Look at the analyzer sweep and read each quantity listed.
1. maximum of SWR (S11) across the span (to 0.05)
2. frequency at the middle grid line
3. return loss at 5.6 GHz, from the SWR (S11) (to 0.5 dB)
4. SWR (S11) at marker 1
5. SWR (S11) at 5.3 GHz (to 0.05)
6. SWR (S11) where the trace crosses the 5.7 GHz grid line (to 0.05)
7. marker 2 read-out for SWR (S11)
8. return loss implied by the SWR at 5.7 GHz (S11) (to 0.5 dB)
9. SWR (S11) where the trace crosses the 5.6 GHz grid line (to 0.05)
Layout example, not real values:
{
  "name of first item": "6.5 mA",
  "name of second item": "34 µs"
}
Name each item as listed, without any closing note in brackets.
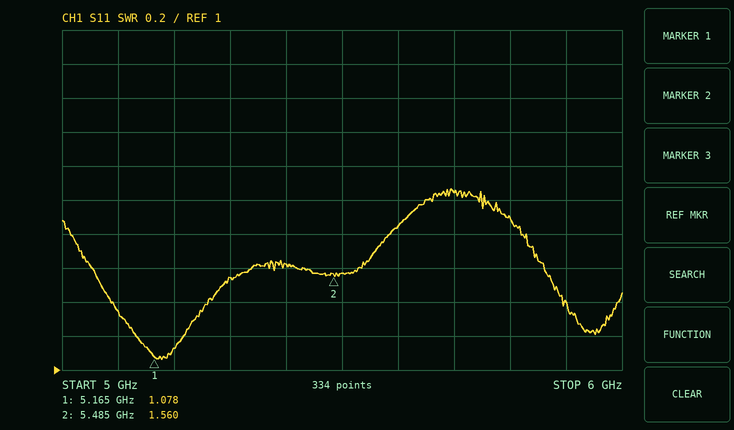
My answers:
{
  "maximum of SWR (S11) across the span": "2.05",
  "frequency at the middle grid line": "5.5 GHz",
  "return loss at 5.6 GHz, from the SWR (S11)": "10.5 dB",
  "SWR (S11) at marker 1": "1.078",
  "SWR (S11) at 5.3 GHz": "1.55",
  "SWR (S11) where the trace crosses the 5.7 GHz grid line": "2.05",
  "marker 2 read-out for SWR": "1.560",
  "return loss implied by the SWR at 5.7 GHz (S11)": "9.5 dB",
  "SWR (S11) where the trace crosses the 5.6 GHz grid line": "1.85"
}
